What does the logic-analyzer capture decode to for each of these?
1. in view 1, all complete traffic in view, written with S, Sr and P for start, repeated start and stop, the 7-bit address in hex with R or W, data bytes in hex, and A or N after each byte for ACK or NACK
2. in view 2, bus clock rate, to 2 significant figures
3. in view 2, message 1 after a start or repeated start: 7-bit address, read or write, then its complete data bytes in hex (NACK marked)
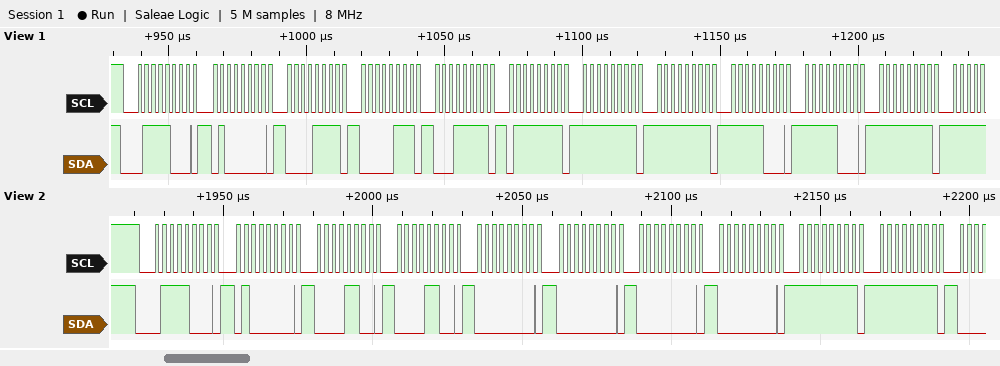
S 3CW A 40 A 0F A 07 A 1F A 7F A FF A FF A F8 A F8 A FF A
400 kHz
0x3C write: 40 0C 0C 00 00 00 00 FF FF
